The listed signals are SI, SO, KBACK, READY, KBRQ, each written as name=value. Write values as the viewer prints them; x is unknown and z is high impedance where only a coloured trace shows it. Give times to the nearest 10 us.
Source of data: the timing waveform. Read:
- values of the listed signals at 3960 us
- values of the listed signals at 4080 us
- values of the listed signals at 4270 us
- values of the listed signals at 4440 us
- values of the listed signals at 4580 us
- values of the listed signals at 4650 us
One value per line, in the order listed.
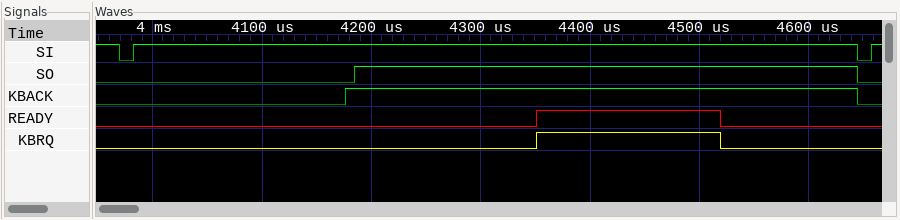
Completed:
SI=1, SO=0, KBACK=0, READY=0, KBRQ=0
SI=1, SO=0, KBACK=0, READY=0, KBRQ=0
SI=1, SO=1, KBACK=1, READY=0, KBRQ=0
SI=1, SO=1, KBACK=1, READY=1, KBRQ=1
SI=1, SO=1, KBACK=1, READY=0, KBRQ=0
SI=0, SO=0, KBACK=0, READY=0, KBRQ=0
